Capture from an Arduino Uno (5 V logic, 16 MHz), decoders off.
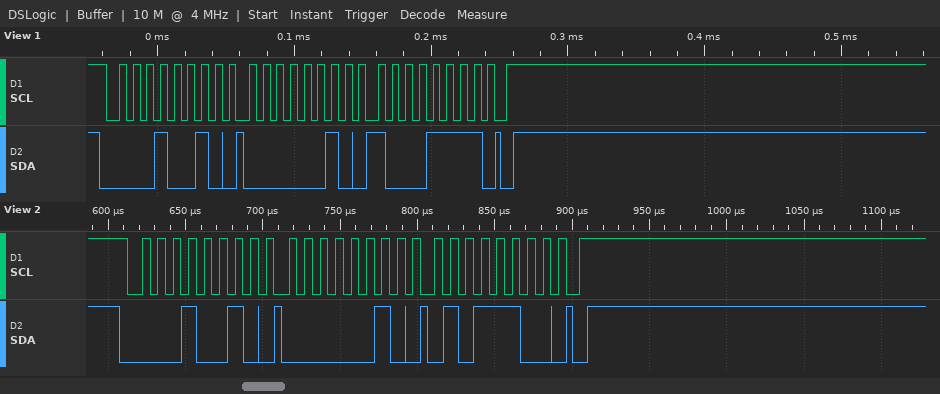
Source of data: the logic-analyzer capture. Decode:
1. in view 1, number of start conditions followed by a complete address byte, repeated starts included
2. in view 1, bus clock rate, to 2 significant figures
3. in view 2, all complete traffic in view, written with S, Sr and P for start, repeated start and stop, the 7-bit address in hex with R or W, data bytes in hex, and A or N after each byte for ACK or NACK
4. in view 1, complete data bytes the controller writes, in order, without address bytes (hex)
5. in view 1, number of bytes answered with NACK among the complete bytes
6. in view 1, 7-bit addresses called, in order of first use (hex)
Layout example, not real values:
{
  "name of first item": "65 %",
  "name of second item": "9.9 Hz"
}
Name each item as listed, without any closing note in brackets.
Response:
{
  "in view 1, number of start conditions followed by a complete address byte, repeated starts included": "1",
  "in view 1, bus clock rate, to 2 significant figures": "100 kHz",
  "in view 2, all complete traffic in view, written with S, Sr and P for start, repeated start and stop, the 7-bit address in hex with R or W, data bytes in hex, and A or N after each byte for ACK or NACK": "S 09W A 02 A 5C A P",
  "in view 1, complete data bytes the controller writes, in order, without address bytes": "02 8F",
  "in view 1, number of bytes answered with NACK among the complete bytes": "0",
  "in view 1, 7-bit addresses called, in order of first use": "0x09"
}
